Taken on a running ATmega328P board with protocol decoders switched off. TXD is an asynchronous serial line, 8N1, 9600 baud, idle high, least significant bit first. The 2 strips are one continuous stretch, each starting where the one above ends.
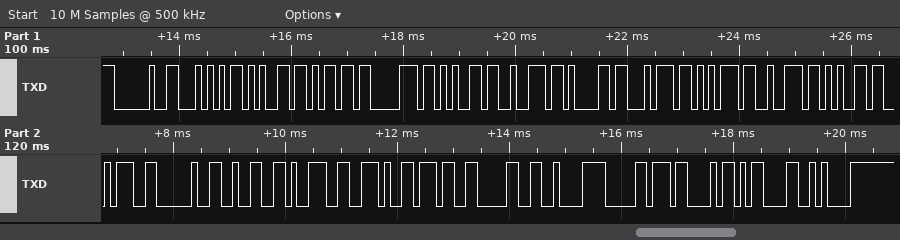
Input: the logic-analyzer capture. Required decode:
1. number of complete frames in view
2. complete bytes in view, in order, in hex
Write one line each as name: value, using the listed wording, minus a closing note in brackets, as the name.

number of complete frames in view: 24
complete bytes in view, in order, in hex: 0x20 0x54 0x65 0x6D 0x70 0x65 0x72 0x61 0x74 0x75 0x72 0x65 0x3A 0x20 0x32 0x39 0x2E 0x37 0x30 0xC2 0xB0 0x43 0x0D 0x0A
